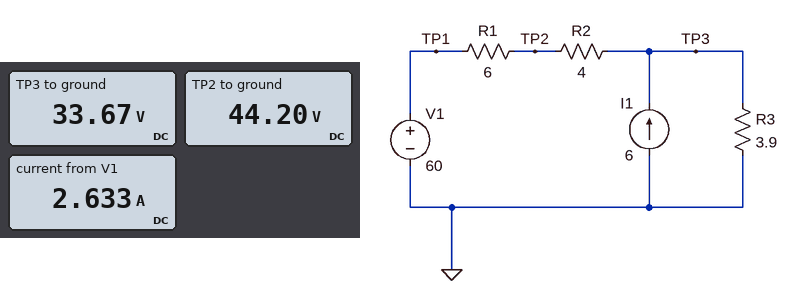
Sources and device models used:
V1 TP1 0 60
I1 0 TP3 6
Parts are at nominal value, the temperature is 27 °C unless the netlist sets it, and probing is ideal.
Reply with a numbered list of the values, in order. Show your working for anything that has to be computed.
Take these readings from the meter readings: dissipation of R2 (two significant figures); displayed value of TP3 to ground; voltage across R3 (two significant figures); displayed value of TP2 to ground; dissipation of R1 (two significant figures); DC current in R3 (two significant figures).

1. (44.2 V - 33.67 V)^2 / 4 Ω = 28 W
2. 33.67 V
3. 33.67 V = 34 V
4. 44.20 V
5. (60 V - 44.2 V)^2 / 6 Ω = 42 W
6. (33.67 V) / 3.9 Ω = 8.6 A
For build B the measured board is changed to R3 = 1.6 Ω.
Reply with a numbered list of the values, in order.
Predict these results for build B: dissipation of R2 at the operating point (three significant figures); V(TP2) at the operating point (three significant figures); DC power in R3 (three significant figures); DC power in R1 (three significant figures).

1. 75.5 W
2. 33.9 V
3. 171 W
4. 113 W
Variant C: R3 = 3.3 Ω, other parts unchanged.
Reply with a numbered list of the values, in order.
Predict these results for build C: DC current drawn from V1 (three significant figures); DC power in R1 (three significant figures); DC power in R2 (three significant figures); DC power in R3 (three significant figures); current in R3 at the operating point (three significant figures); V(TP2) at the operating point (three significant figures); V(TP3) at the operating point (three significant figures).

1. 3.02 A
2. 54.8 W
3. 36.5 W
4. 269 W
5. 9.02 A
6. 41.9 V
7. 29.8 V
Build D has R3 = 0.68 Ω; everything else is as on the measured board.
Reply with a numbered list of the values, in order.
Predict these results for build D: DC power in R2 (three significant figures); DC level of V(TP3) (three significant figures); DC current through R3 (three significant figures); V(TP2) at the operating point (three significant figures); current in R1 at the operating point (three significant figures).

1. 110 W
2. 7.64 V
3. 11.2 A
4. 28.6 V
5. 5.24 A
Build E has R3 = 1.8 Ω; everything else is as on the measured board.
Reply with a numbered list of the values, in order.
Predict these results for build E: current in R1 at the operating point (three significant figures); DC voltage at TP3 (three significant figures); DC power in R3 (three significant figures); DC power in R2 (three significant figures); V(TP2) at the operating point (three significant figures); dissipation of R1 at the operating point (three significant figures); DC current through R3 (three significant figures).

1. 4.17 A
2. 18.3 V
3. 186 W
4. 69.5 W
5. 35.0 V
6. 104 W
7. 10.2 A
